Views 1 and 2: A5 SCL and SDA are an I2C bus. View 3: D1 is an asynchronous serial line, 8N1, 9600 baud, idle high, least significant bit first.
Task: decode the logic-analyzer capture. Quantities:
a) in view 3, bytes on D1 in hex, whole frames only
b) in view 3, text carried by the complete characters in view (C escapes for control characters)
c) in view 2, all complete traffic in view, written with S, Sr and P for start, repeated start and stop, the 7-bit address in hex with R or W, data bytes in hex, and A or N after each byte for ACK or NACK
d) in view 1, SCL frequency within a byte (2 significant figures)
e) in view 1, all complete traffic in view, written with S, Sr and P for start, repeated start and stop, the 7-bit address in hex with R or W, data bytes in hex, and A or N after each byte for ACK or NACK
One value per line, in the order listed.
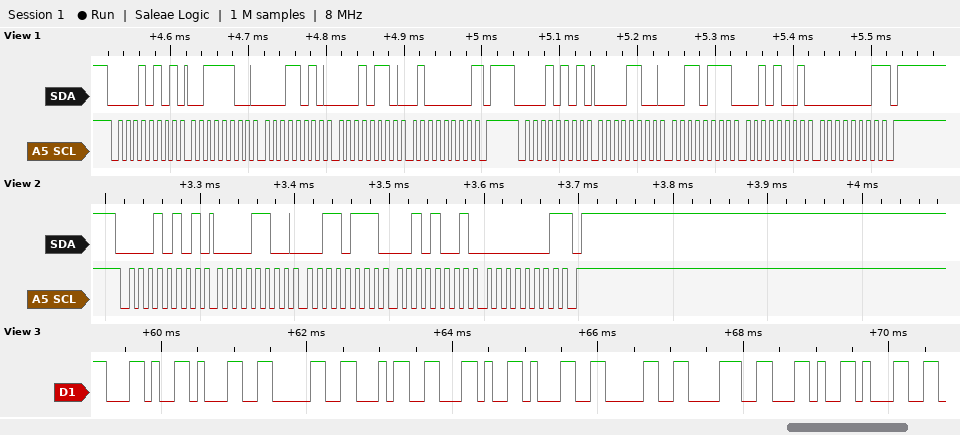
2C 31 30 34 2C 31 30 38 2C 31
",104,108,1"
S 0AR A 0C A 37 A 29 A 01 N P
100 kHz
S 0AR A 3C A 1A A 16 A 40 N P S 0AR A 0C A 37 A 29 A 01 N P
